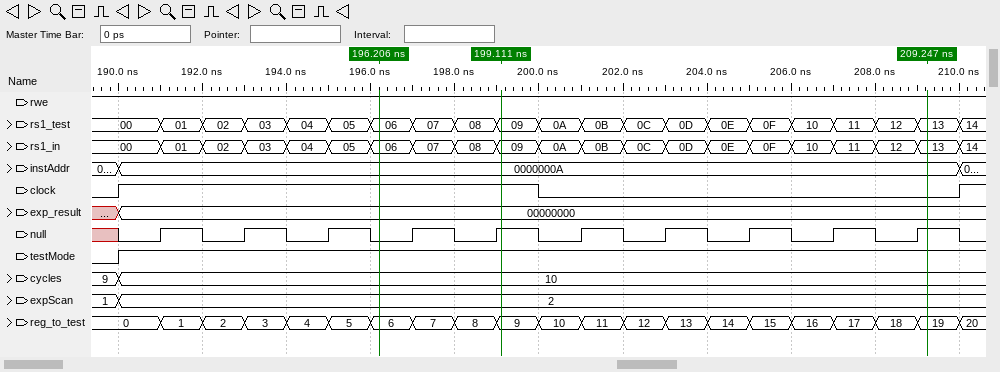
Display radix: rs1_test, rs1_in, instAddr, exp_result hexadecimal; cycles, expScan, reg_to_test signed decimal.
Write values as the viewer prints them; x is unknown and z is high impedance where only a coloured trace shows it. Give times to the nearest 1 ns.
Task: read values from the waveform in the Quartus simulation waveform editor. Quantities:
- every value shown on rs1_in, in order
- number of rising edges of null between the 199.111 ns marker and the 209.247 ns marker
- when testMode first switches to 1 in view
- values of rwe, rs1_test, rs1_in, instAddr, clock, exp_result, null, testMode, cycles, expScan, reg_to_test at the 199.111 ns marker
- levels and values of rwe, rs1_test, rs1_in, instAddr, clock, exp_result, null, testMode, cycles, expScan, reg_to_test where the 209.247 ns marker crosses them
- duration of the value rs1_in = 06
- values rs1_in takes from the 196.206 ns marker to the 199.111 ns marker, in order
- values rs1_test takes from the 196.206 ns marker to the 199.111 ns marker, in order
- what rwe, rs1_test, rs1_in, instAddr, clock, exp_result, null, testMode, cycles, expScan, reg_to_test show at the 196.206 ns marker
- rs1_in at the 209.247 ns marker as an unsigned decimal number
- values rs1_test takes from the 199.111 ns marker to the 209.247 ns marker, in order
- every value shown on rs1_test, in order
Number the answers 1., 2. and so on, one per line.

1. 00, 01, 02, 03, 04, 05, 06, 07, 08, 09, 0A, 0B, 0C, 0D, 0E, 0F, 10, 11, 12, 13, 14
2. 5
3. 190 ns
4. rwe=1, rs1_test=09, rs1_in=09, instAddr=0000000A, clock=1, exp_result=00000000, null=1, testMode=1, cycles=10, expScan=2, reg_to_test=9
5. rwe=1, rs1_test=13, rs1_in=13, instAddr=0000000A, clock=0, exp_result=00000000, null=1, testMode=1, cycles=10, expScan=2, reg_to_test=19
6. 1 ns
7. 06, 07, 08, 09
8. 06, 07, 08, 09
9. rwe=1, rs1_test=06, rs1_in=06, instAddr=0000000A, clock=1, exp_result=00000000, null=0, testMode=1, cycles=10, expScan=2, reg_to_test=6
10. 19
11. 09, 0A, 0B, 0C, 0D, 0E, 0F, 10, 11, 12, 13
12. 00, 01, 02, 03, 04, 05, 06, 07, 08, 09, 0A, 0B, 0C, 0D, 0E, 0F, 10, 11, 12, 13, 14
